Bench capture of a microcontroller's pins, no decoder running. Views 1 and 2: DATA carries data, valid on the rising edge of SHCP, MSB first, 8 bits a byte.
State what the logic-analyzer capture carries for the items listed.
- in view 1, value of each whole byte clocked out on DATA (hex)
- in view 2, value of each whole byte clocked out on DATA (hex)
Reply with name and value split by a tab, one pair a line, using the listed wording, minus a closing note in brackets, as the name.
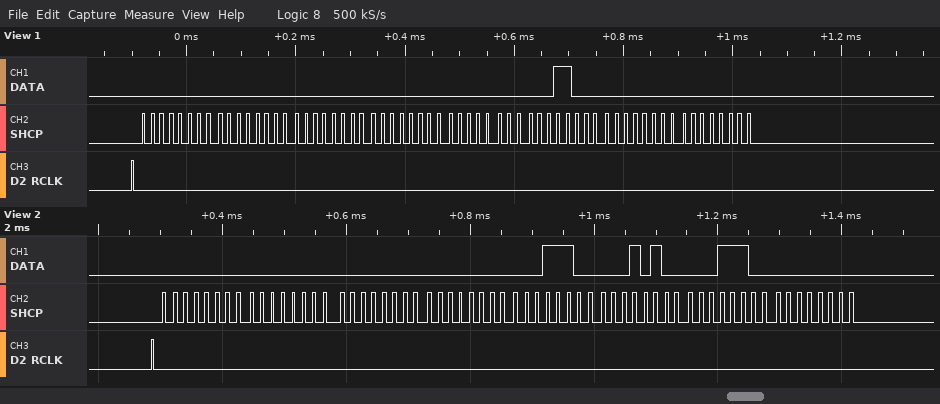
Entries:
in view 1, value of each whole byte clocked out on DATA	00 00 00 00 00 18 00 00
in view 2, value of each whole byte clocked out on DATA	00 00 00 00 1C 14 1C 00
